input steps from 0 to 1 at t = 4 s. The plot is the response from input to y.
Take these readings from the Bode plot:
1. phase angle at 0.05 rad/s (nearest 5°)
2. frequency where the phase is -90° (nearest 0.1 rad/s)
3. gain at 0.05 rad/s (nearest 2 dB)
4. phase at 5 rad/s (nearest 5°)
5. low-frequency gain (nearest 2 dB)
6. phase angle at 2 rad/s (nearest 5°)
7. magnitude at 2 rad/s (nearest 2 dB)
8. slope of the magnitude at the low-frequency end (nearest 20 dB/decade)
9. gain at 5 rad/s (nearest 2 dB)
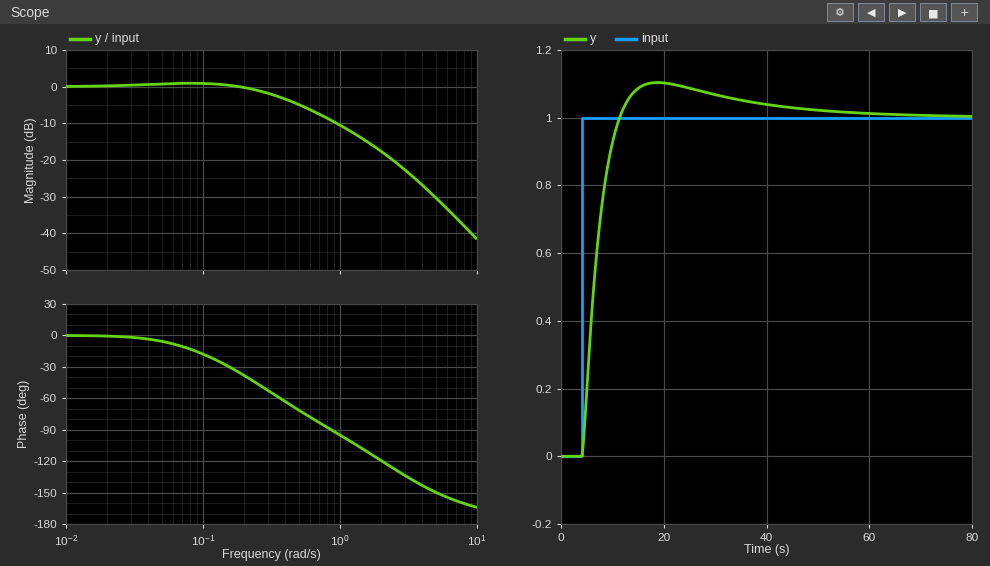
-5°
0.9 rad/s
0 dB
-150°
0 dB
-120°
-18 dB
0 dB/decade
-30 dB
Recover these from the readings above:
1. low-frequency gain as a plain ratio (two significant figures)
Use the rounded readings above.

1.0
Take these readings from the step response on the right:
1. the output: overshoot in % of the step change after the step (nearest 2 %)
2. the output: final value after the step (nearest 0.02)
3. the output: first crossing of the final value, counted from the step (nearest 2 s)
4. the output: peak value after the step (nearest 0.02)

10 %
1.00
8 s
1.10
